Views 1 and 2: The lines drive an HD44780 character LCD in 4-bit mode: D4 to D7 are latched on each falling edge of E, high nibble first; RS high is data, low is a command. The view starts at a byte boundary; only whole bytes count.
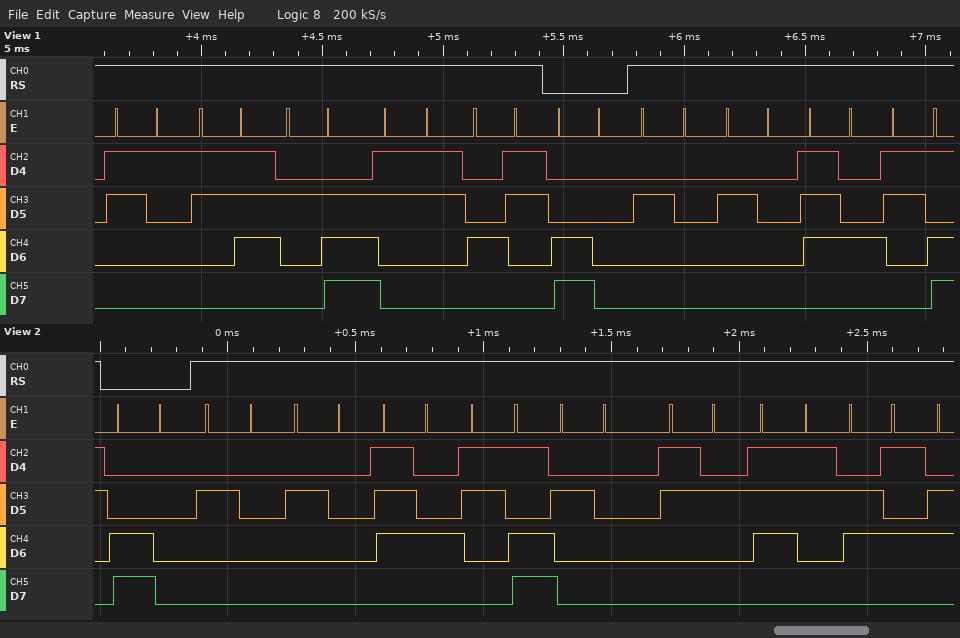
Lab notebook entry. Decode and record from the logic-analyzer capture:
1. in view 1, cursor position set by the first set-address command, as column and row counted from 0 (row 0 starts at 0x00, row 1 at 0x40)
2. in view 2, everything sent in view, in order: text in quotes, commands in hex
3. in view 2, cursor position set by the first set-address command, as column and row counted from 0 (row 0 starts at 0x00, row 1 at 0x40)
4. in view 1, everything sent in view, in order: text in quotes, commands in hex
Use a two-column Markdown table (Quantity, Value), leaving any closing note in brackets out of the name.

| Quantity | Value |
|---|---|
| in view 1, cursor position set by the first set-address command, as column and row counted from 0 | column 0, row 1 |
| in view 2, everything sent in view, in order: text in quotes, commands in hex | 0xC0 "  t= 2se" |
| in view 2, cursor position set by the first set-address command, as column and row counted from 0 | column 0, row 1 |
| in view 1, everything sent in view, in order: text in quotes, commands in hex | "17.3C" 0xC0 "  t=" |
